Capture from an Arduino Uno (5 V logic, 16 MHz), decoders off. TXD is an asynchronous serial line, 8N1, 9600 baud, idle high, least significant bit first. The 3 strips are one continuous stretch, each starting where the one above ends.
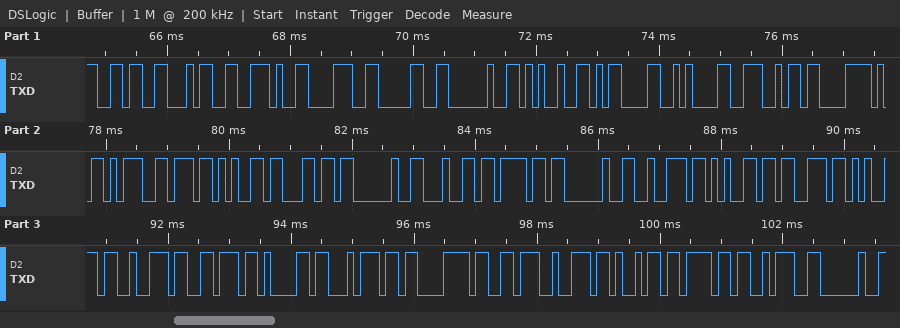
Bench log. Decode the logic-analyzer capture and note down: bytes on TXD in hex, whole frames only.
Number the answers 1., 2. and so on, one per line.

1. 36 34 2E 38 30 20 25 0D 0A 4E C3 AD 76 65 6C 20 64 6F 20 72 65 73 65 72 76 61 74 C3 B3 72 69 6F 3A 20
